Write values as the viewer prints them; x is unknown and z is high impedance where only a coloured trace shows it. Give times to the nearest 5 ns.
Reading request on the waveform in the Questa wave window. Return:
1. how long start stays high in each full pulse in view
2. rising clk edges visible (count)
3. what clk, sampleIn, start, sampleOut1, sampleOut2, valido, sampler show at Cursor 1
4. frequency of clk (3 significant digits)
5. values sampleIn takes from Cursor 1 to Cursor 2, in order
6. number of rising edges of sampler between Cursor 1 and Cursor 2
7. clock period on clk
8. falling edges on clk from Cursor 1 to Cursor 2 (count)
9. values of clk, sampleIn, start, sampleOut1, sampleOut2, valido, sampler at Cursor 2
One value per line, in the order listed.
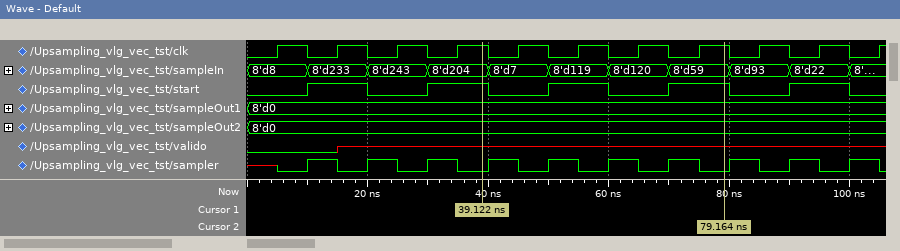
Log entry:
10 ns, 10 ns, 10 ns, 10 ns, 10 ns
11
clk=1, sampleIn=8'd204, start=1, sampleOut1=8'd0, sampleOut2=8'd0, valido=x, sampler=0
100 MHz
8'd204, 8'd7, 8'd119, 8'd120, 8'd59
4
10 ns
4
clk=1, sampleIn=8'd59, start=1, sampleOut1=8'd0, sampleOut2=8'd0, valido=x, sampler=0
